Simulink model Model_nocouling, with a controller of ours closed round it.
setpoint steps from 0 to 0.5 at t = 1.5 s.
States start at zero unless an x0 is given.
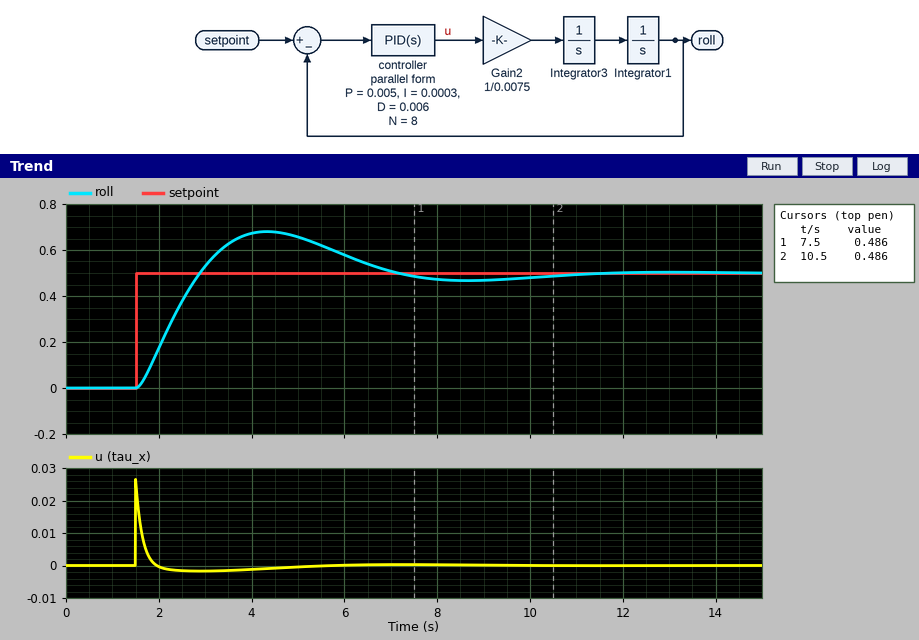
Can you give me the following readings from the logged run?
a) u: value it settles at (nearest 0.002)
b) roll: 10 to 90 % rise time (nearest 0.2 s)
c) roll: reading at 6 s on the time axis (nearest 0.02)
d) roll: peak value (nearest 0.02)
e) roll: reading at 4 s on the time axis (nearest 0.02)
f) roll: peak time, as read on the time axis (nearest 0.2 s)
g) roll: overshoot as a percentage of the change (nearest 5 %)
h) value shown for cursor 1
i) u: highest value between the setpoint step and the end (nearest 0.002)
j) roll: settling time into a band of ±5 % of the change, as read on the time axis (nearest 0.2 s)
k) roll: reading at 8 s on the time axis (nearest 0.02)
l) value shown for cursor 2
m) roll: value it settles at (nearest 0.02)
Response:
0.000
1.0 s
0.58
0.68
0.68
4.4 s
35 %
0.486
0.026
9.6 s
0.48
0.486
0.50
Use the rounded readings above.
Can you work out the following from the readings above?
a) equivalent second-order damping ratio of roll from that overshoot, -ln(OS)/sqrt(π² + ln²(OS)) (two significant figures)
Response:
0.32
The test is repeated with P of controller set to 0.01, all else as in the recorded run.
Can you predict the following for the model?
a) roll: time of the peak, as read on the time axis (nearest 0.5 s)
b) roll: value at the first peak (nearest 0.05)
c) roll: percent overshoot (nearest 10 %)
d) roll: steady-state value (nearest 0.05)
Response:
3.5 s
0.75
50 %
0.50
